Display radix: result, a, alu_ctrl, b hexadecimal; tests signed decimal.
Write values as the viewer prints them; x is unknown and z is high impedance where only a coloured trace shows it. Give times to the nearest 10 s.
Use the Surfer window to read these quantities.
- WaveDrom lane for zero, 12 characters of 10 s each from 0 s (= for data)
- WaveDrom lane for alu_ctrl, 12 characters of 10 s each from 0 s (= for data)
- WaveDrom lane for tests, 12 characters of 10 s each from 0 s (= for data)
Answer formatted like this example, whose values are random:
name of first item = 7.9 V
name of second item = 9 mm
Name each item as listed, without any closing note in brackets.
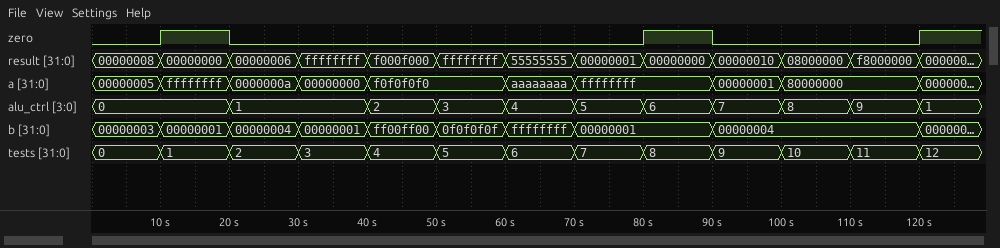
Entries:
WaveDrom lane for zero, 12 characters of 10 s each from 0 s = {name: 'zero', wave: '010.....10..'}
WaveDrom lane for alu_ctrl, 12 characters of 10 s each from 0 s = {name: 'alu_ctrl', wave: '=.=.========', data: '0 1 2 3 4 5 6 7 8 9'}
WaveDrom lane for tests, 12 characters of 10 s each from 0 s = {name: 'tests', wave: '============', data: '0 1 2 3 4 5 6 7 8 9 10 11'}
